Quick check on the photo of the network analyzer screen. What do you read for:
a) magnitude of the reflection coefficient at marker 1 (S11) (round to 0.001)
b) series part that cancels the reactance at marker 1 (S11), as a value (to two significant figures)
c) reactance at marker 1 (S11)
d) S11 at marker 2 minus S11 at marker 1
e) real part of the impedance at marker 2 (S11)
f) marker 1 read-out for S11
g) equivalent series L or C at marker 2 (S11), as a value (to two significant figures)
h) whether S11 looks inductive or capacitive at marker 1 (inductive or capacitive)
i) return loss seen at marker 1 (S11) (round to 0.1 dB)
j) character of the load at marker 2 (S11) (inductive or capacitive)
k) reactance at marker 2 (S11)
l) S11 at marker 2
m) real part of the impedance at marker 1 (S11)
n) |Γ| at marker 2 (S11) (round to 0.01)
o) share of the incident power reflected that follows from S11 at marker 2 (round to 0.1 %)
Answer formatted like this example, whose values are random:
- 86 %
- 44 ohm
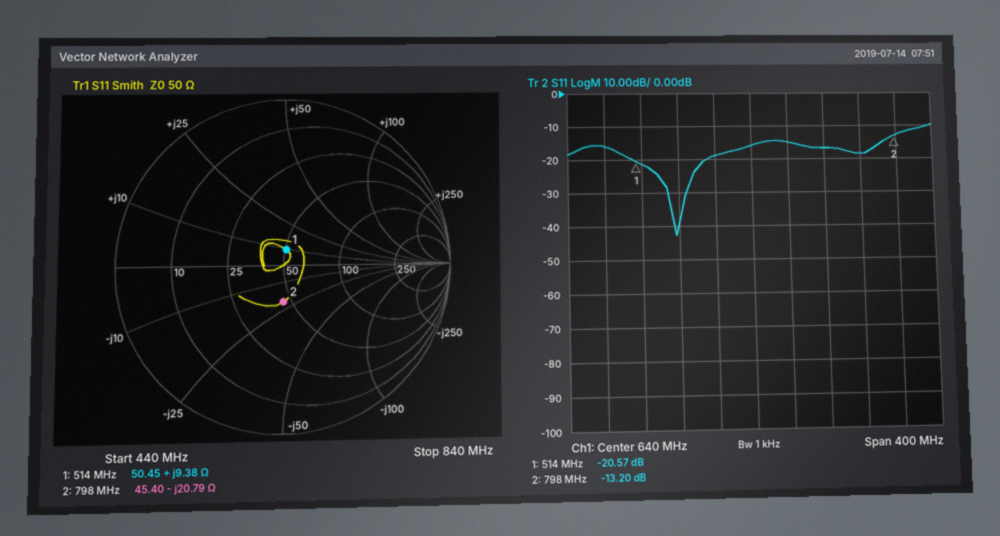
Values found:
- 0.094
- 33 pF
- +9.38 Ω
- 7.37 dB
- 45.40 Ω
- -20.57 dB
- 9.6 pF
- inductive
- 20.6 dB
- capacitive
- -20.79 Ω
- -13.20 dB
- 50.45 Ω
- 0.22
- 4.8 %
